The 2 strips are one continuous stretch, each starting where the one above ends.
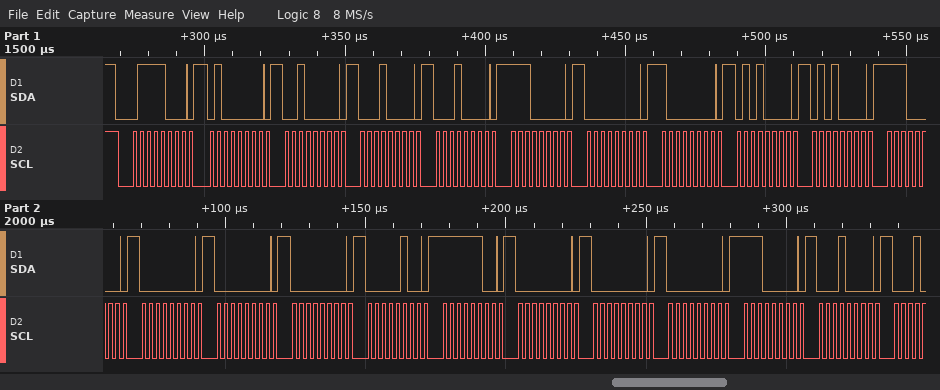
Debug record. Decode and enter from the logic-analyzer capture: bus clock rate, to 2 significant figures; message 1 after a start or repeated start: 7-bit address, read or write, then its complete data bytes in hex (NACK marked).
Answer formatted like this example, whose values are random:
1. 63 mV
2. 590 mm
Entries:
1. 400 kHz
2. 0x3C write: 40 20 10 10 E0 00 80 50 50 E0 00 00 00 04 FC 00 00 00 E0 10
